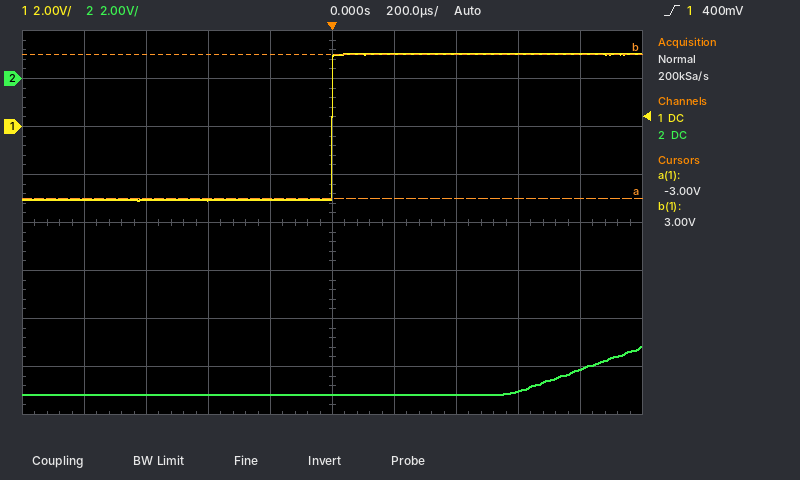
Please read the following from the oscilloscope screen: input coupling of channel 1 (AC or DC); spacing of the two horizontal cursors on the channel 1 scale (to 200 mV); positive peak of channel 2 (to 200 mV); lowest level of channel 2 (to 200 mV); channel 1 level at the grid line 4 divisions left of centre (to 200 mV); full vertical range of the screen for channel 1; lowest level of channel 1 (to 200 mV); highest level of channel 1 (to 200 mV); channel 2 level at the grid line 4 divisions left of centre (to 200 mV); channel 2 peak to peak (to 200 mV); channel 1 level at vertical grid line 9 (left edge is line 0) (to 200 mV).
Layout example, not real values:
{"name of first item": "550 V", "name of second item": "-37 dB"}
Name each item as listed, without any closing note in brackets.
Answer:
{"input coupling of channel 1": "DC", "spacing of the two horizontal cursors on the channel 1 scale": "6.0 V", "positive peak of channel 2": "-11.2 V", "lowest level of channel 2": "-13.2 V", "channel 1 level at the grid line 4 divisions left of centre": "-3.0 V", "full vertical range of the screen for channel 1": "16 V", "lowest level of channel 1": "-3.0 V", "highest level of channel 1": "3.0 V", "channel 2 level at the grid line 4 divisions left of centre": "-13.2 V", "channel 2 peak to peak": "2.0 V", "channel 1 level at vertical grid line 9 (left edge is line 0)": "3.0 V"}
